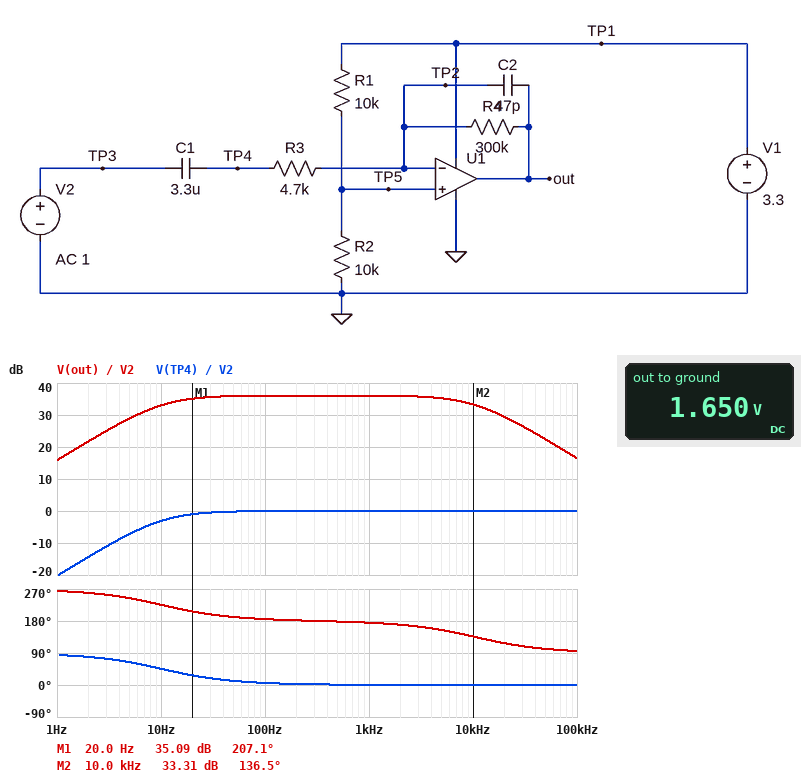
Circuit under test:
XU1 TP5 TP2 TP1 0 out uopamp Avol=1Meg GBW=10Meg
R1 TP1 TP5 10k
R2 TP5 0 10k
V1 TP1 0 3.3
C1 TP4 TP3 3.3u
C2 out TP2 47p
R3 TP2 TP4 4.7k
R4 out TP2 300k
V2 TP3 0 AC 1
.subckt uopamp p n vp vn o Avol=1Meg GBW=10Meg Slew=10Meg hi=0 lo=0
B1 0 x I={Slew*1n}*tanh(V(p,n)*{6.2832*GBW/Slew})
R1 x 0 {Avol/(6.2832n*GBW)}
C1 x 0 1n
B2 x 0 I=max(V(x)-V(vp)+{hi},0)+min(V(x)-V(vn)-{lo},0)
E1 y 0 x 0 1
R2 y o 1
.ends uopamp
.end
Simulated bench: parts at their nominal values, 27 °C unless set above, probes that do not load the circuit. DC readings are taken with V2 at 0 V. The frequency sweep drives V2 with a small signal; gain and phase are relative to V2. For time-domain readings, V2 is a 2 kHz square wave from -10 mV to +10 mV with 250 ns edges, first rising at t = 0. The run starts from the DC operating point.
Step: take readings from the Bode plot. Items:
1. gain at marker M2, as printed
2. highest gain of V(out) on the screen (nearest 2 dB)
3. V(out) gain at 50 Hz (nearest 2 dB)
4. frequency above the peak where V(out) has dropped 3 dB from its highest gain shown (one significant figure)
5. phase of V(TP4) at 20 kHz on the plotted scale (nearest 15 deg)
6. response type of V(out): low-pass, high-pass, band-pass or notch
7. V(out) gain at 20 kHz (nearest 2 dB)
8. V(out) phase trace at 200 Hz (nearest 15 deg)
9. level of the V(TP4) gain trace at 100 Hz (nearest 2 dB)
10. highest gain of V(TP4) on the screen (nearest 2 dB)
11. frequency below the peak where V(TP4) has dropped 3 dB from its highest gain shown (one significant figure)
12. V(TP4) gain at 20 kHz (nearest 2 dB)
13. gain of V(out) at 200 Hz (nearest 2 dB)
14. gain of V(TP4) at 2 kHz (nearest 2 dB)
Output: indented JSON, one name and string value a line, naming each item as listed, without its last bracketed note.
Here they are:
{
  "gain at marker M2, as printed": "33.31 dB",
  "highest gain of V(out) on the screen": "36 dB",
  "V(out) gain at 50 Hz": "36 dB",
  "frequency above the peak where V(out) has dropped 3 dB from its highest gain shown": "10 kHz",
  "phase of V(TP4) at 20 kHz on the plotted scale": "0 deg",
  "response type of V(out): low-pass, high-pass, band-pass or notch": "band-pass",
  "V(out) gain at 20 kHz": "30 dB",
  "V(out) phase trace at 200 Hz": "180 deg",
  "level of the V(TP4) gain trace at 100 Hz": "0 dB",
  "highest gain of V(TP4) on the screen": "0 dB",
  "frequency below the peak where V(TP4) has dropped 3 dB from its highest gain shown": "10 Hz",
  "V(TP4) gain at 20 kHz": "0 dB",
  "gain of V(out) at 200 Hz": "36 dB",
  "gain of V(TP4) at 2 kHz": "0 dB"
}
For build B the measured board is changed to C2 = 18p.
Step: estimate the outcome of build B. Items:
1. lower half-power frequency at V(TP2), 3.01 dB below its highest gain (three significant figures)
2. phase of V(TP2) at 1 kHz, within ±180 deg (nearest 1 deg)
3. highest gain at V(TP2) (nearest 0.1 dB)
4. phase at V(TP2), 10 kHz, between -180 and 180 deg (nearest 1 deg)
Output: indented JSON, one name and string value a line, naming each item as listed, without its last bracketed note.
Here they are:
{
  "lower half-power frequency at V(TP2), 3.01 dB below its highest gain": "24.7 kHz",
  "phase of V(TP2) at 1 kHz, within ±180 deg": "88 deg",
  "highest gain at V(TP2)": "-16.0 dB",
  "phase at V(TP2), 10 kHz, between -180 and 180 deg": "68 deg"
}
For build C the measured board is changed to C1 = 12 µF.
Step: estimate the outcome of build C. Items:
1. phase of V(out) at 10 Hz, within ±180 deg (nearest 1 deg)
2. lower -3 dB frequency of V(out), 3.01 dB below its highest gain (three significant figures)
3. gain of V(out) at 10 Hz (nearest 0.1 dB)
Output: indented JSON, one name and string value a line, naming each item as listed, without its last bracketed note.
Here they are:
{
  "phase of V(out) at 10 Hz, within ±180 deg": "-164 deg",
  "lower -3 dB frequency of V(out), 3.01 dB below its highest gain": "2.82 Hz",
  "gain of V(out) at 10 Hz": "35.8 dB"
}
